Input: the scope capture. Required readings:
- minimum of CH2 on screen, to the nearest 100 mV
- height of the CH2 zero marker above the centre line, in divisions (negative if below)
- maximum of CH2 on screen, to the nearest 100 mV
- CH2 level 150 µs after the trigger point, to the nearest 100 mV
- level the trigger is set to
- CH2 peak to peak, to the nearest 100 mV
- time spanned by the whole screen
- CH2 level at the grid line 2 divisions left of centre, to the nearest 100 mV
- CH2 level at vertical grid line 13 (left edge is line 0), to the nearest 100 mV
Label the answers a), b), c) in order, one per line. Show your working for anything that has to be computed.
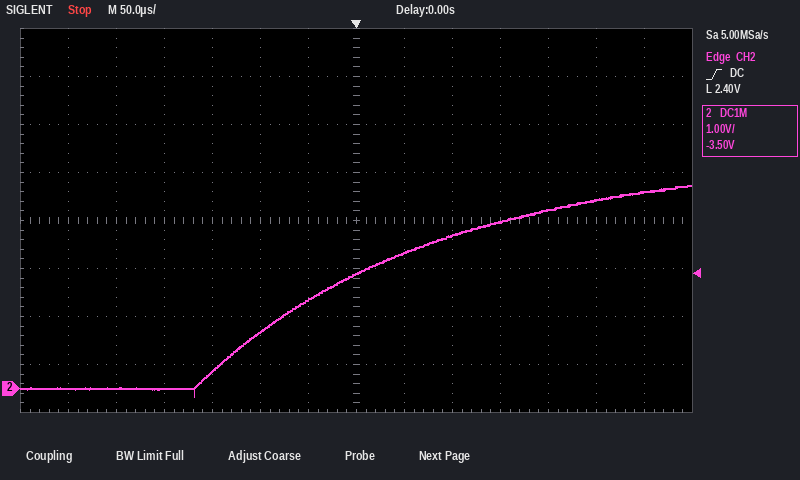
a) -200 mV
b) -3.5 div
c) 4.2 V
d) 3.5 V
e) 2.40 V
f) 4.2 V − (-200 mV) = 4.4 V
g) 700 µs
h) 1.2 V
i) 4.1 V
